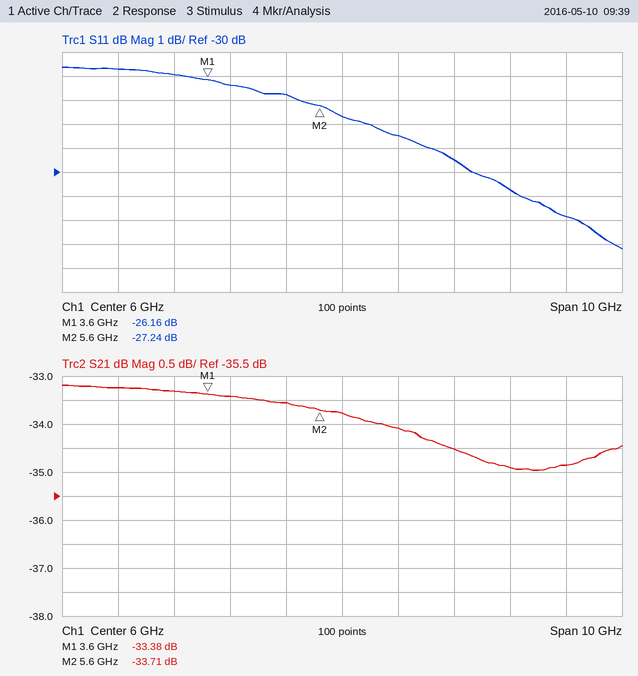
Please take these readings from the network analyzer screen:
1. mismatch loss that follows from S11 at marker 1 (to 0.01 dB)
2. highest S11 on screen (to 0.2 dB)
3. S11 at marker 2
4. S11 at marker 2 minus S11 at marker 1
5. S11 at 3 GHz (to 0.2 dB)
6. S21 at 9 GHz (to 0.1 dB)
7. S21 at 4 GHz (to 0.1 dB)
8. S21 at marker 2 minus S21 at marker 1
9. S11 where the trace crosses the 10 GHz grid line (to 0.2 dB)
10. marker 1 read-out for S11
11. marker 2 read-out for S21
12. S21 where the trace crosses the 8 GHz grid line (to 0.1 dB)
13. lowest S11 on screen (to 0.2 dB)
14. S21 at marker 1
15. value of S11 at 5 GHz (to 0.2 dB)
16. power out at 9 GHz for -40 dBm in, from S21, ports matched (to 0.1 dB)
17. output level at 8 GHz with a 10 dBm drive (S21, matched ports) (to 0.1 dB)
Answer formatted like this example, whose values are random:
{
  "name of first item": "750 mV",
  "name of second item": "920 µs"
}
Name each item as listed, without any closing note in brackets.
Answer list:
{
  "mismatch loss that follows from S11 at marker 1": "0.01 dB",
  "highest S11 on screen": "-25.6 dB",
  "S11 at marker 2": "-27.24 dB",
  "S11 at marker 2 minus S11 at marker 1": "-1.08 dB",
  "S11 at 3 GHz": "-26.0 dB",
  "S21 at 9 GHz": "-34.9 dB",
  "S21 at 4 GHz": "-33.4 dB",
  "S21 at marker 2 minus S21 at marker 1": "-0.33 dB",
  "S11 where the trace crosses the 10 GHz grid line": "-31.8 dB",
  "marker 1 read-out for S11": "-26.16 dB",
  "marker 2 read-out for S21": "-33.71 dB",
  "S21 where the trace crosses the 8 GHz grid line": "-34.5 dB",
  "lowest S11 on screen": "-33.2 dB",
  "S21 at marker 1": "-33.38 dB",
  "value of S11 at 5 GHz": "-26.8 dB",
  "power out at 9 GHz for -40 dBm in, from S21, ports matched": "-74.9 dBm",
  "output level at 8 GHz with a 10 dBm drive (S21, matched ports)": "-24.5 dBm"
}
